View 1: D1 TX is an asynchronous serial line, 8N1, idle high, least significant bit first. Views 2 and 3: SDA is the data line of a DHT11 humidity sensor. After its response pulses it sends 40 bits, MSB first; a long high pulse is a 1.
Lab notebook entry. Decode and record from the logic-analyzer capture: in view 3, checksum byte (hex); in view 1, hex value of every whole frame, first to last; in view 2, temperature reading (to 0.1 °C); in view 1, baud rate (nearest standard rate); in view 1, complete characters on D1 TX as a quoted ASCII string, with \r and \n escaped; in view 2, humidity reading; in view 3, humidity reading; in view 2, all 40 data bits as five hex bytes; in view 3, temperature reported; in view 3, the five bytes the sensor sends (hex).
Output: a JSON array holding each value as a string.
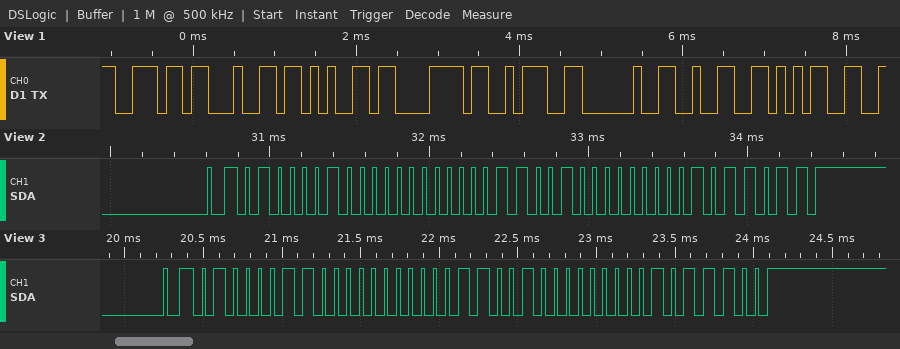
["0x5C", "6E 64 65 78 3A 20 32 35", "25.0 °C", "9600 baud", "\"ndex: 25\"", "66 %", "67 %", "42 00 19 00 5B", "25.0 °C", "43 00 19 00 5C"]
